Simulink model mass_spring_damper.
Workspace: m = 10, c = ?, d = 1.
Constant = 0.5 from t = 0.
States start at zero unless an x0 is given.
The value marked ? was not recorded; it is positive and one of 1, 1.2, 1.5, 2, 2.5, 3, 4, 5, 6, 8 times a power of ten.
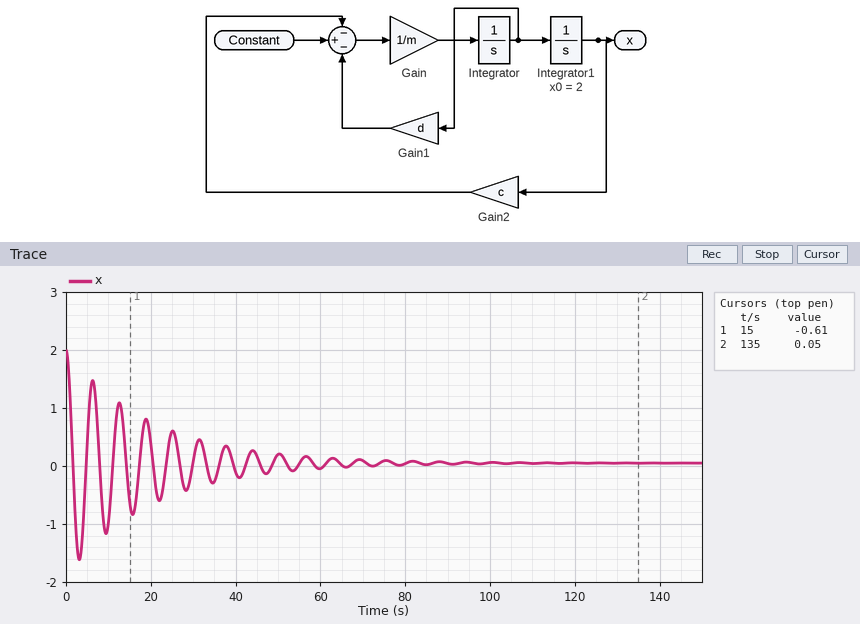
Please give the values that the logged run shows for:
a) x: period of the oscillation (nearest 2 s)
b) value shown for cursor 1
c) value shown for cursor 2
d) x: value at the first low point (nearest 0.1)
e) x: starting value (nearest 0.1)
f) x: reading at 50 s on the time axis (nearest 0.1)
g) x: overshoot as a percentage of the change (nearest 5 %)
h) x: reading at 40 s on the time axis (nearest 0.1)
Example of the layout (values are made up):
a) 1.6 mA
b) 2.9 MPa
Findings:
a) 6 s
b) -0.61
c) 0.05
d) -1.6
e) 2.0
f) 0.2
g) 85 %
h) -0.1
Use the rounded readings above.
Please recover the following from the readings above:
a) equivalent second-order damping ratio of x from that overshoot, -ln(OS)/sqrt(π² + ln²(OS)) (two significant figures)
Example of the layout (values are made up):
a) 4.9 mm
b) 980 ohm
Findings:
a) 0.052
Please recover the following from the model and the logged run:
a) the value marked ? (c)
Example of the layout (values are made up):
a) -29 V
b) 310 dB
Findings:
a) 10
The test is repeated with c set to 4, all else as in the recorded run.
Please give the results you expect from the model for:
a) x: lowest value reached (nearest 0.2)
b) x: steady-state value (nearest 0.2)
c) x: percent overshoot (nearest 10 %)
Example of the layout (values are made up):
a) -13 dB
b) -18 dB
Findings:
a) -1.4
b) 0.2
c) 80 %
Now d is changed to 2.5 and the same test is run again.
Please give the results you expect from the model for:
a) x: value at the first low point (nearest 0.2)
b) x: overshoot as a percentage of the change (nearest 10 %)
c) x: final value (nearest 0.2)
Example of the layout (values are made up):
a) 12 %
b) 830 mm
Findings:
a) -1.2
b) 70 %
c) 0.0
